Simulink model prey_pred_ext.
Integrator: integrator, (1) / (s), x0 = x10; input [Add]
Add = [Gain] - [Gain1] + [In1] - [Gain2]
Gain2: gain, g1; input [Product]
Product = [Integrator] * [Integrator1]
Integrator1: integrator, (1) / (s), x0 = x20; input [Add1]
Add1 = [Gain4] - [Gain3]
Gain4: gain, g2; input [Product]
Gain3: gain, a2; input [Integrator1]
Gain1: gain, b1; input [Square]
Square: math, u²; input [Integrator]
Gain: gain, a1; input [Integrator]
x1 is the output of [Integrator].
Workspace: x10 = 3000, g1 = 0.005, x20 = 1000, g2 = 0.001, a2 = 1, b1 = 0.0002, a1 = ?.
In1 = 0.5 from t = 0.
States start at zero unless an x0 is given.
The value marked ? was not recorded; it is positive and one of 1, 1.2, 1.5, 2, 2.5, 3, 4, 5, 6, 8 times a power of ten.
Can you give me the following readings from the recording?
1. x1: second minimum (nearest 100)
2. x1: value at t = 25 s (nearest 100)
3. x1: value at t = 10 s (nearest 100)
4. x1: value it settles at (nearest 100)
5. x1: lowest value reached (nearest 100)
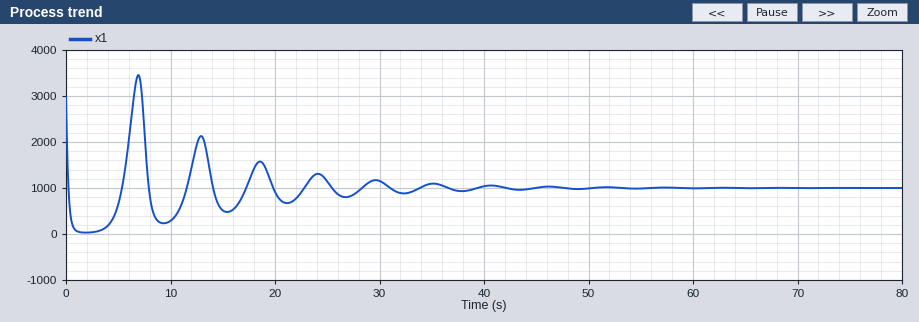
200
1100
300
1000
0
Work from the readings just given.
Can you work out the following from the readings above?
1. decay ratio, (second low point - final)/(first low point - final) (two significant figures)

0.80
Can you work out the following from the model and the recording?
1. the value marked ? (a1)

1.5
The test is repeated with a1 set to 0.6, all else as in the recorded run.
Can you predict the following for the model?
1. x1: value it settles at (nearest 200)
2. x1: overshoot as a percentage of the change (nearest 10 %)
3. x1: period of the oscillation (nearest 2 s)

1000
50 %
20 s
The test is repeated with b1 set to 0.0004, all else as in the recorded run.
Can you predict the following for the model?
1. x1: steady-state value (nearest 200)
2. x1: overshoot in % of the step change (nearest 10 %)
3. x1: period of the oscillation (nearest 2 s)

1000
50 %
8 s
